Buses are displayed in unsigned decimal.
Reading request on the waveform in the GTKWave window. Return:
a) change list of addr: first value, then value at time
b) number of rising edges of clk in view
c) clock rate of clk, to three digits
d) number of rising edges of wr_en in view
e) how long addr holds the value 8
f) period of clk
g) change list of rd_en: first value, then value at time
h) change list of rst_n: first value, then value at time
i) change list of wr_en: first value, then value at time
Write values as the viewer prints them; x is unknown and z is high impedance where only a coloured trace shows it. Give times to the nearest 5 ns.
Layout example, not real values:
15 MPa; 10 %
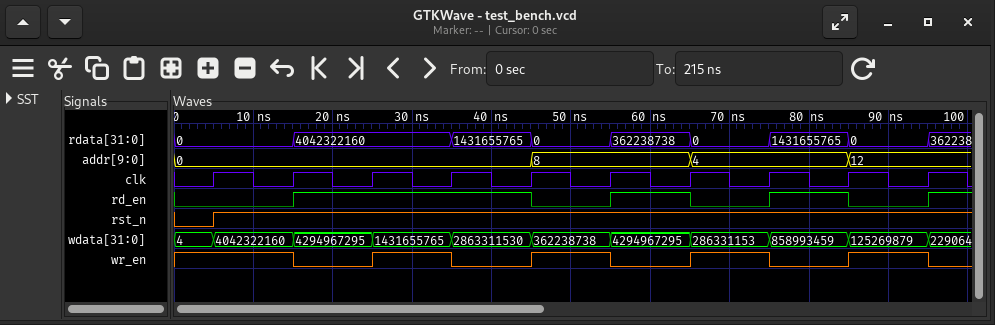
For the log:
0, 8 at 45 ns, 4 at 65 ns, 12 at 85 ns; 10; 100 MHz; 4; 20 ns; 10 ns; 0, 1 at 15 ns, 0 at 45 ns, 1 at 55 ns, 0 at 65 ns, 1 at 75 ns, 0 at 85 ns, 1 at 95 ns; 0, 1 at 5 ns; 1, 0 at 15 ns, 1 at 25 ns, 0 at 35 ns, 1 at 45 ns, 0 at 55 ns, 1 at 65 ns, 0 at 75 ns, 1 at 85 ns, 0 at 95 ns
